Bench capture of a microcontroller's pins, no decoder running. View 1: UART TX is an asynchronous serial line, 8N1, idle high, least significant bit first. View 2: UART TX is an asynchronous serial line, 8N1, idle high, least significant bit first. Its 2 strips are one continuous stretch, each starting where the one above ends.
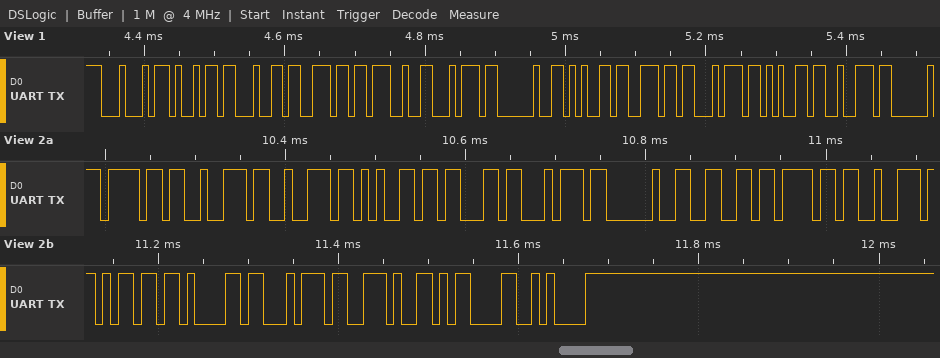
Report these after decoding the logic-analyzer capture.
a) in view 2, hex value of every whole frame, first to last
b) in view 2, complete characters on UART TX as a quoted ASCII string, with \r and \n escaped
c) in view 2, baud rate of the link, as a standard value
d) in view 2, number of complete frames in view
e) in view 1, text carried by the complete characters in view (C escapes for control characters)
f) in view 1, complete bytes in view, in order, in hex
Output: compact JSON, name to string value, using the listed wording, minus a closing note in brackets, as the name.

{"in view 2, hex value of every whole frame, first to last": "0x6F 0x72 0x72 0x65 0x63 0x74 0x20 0x66 0x6F 0x72 0x6D 0x61 0x74 0x2E 0x0D 0x0A", "in view 2, complete characters on UART TX as a quoted ASCII string, with \\r and \\n escaped": "\"orrect format.\\r\\n\"", "in view 2, baud rate of the link, as a standard value": "115200 baud", "in view 2, number of complete frames in view": "16", "in view 1, text carried by the complete characters in view": "\"Didn't enter\"", "in view 1, complete bytes in view, in order, in hex": "44 69 64 6E 27 74 20 65 6E 74 65 72"}
